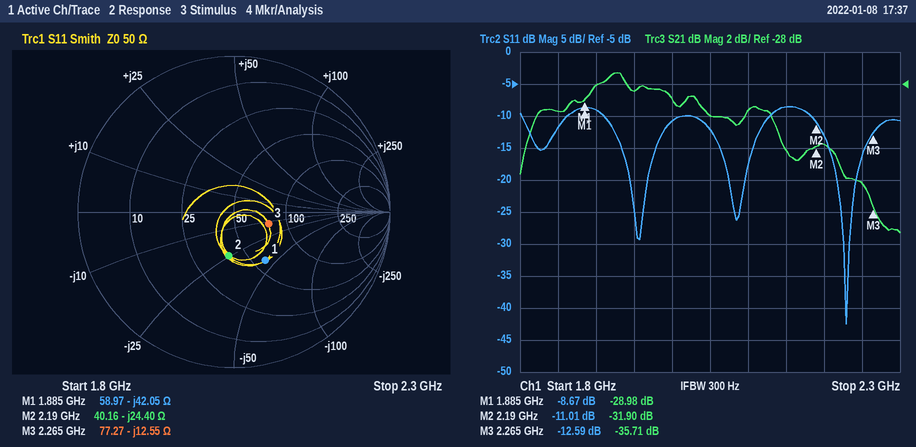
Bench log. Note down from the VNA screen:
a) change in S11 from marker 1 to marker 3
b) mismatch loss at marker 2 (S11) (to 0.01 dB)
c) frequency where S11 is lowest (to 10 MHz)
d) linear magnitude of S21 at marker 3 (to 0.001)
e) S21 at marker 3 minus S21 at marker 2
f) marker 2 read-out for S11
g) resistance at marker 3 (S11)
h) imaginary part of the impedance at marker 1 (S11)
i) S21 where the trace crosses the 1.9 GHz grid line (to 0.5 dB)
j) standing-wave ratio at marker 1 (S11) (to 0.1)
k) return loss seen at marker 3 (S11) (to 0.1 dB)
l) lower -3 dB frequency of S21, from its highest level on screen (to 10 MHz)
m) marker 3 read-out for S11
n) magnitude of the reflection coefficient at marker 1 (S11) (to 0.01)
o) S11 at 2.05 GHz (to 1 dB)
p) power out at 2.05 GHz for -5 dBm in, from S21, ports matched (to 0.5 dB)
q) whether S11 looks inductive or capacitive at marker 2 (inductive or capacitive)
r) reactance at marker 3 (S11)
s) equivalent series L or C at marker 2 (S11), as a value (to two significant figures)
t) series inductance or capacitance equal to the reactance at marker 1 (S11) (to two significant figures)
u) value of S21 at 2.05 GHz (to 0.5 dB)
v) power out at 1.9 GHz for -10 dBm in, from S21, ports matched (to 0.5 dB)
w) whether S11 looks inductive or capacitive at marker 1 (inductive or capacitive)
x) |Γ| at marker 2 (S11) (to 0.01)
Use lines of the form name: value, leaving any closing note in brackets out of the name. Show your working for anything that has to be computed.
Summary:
change in S11 from marker 1 to marker 3: -12.59 − (-8.67) = -3.92 dB
mismatch loss at marker 2 (S11): −10 log10(1 − 10^(-11.01/10)) ≈ 0.36 dB
frequency where S11 is lowest: 2.23 GHz
linear magnitude of S21 at marker 3: 10^(-35.71/20) ≈ 0.016
S21 at marker 3 minus S21 at marker 2: -35.71 − (-31.9) = -3.81 dB
marker 2 read-out for S11: -11.01 dB
resistance at marker 3: 77.27 Ω
imaginary part of the impedance at marker 1: -42.05 Ω
S21 where the trace crosses the 1.9 GHz grid line: -28.0 dB
standing-wave ratio at marker 1 (S11): 2.2
return loss seen at marker 3 (S11): 12.6 dB
lower -3 dB frequency of S21, from its highest level on screen: 1.82 GHz
marker 3 read-out for S11: -12.59 dB
magnitude of the reflection coefficient at marker 1 (S11): 10^(-8.67/20) ≈ 0.37
S11 at 2.05 GHz: -12 dB
power out at 2.05 GHz for -5 dBm in, from S21, ports matched: -5 dBm + (-30.0 dB) = -35.0 dBm
whether S11 looks inductive or capacitive at marker 2: capacitive
reactance at marker 3: -12.55 Ω
equivalent series L or C at marker 2 (S11), as a value: C = 1/(2π × 2.19 GHz × 24.4 Ω) ≈ 3.0 pF
series inductance or capacitance equal to the reactance at marker 1 (S11): C = 1/(2π × 1.885 GHz × 42.05 Ω) ≈ 2.0 pF
value of S21 at 2.05 GHz: -30.0 dB
power out at 1.9 GHz for -10 dBm in, from S21, ports matched: -10 dBm + (-28.0 dB) = -38.0 dBm
whether S11 looks inductive or capacitive at marker 1: capacitive
|Γ| at marker 2 (S11): 0.28
